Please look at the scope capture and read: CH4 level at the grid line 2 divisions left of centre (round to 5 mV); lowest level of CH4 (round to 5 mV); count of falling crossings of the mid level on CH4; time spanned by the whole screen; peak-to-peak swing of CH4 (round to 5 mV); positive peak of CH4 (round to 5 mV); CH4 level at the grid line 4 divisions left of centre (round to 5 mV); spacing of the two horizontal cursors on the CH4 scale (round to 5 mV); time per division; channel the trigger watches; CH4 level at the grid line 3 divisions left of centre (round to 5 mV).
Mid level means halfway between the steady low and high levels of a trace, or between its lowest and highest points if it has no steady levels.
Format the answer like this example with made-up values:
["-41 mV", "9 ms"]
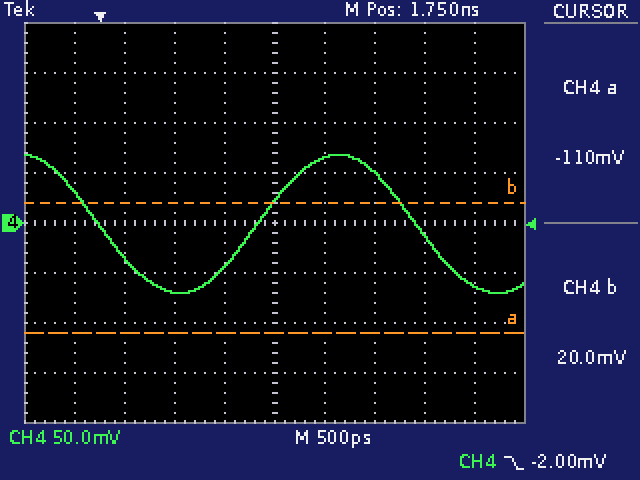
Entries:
["-70 mV", "-70 mV", "2", "5 ns", "140 mV", "70 mV", "30 mV", "130 mV", "500 ps", "CH4", "-35 mV"]
